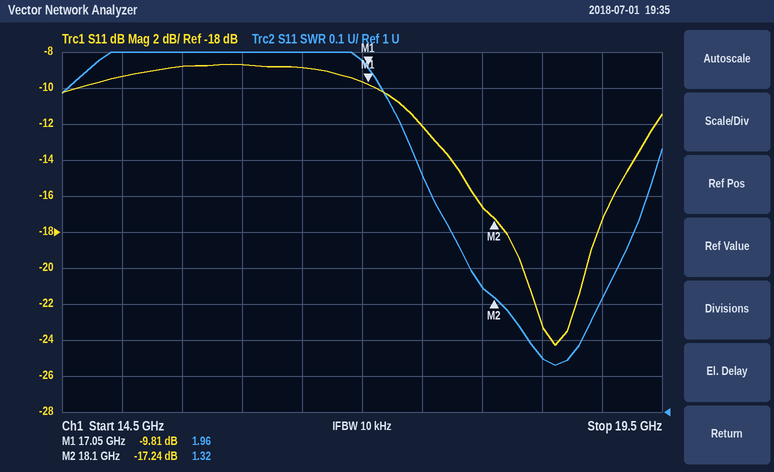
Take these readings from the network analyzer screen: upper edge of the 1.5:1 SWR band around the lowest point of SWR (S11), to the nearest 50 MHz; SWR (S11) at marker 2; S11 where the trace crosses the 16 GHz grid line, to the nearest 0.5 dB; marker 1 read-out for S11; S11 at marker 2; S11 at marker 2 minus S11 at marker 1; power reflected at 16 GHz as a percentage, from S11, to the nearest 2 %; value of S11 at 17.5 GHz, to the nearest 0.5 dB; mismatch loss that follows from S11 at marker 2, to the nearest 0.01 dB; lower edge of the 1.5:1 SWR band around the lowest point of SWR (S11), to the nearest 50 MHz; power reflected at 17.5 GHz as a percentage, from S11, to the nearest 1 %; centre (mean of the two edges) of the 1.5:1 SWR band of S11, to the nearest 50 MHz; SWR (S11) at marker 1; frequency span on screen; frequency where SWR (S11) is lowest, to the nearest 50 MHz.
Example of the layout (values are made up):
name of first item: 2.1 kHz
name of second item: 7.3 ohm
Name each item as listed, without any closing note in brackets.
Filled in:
upper edge of the 1.5:1 SWR band around the lowest point of SWR (S11), to the nearest 50 MHz: 19.25 GHz
SWR (S11) at marker 2: 1.32
S11 where the trace crosses the 16 GHz grid line, to the nearest 0.5 dB: -8.5 dB
marker 1 read-out for S11: -9.81 dB
S11 at marker 2: -17.24 dB
S11 at marker 2 minus S11 at marker 1: -7.43 dB
power reflected at 16 GHz as a percentage, from S11, to the nearest 2 %: 14 %
value of S11 at 17.5 GHz, to the nearest 0.5 dB: -12.0 dB
mismatch loss that follows from S11 at marker 2, to the nearest 0.01 dB: 0.08 dB
lower edge of the 1.5:1 SWR band around the lowest point of SWR (S11), to the nearest 50 MHz: 17.75 GHz
power reflected at 17.5 GHz as a percentage, from S11, to the nearest 1 %: 6 %
centre (mean of the two edges) of the 1.5:1 SWR band of S11, to the nearest 50 MHz: 18.50 GHz
SWR (S11) at marker 1: 1.96
frequency span on screen: 5 GHz
frequency where SWR (S11) is lowest, to the nearest 50 MHz: 18.60 GHz
